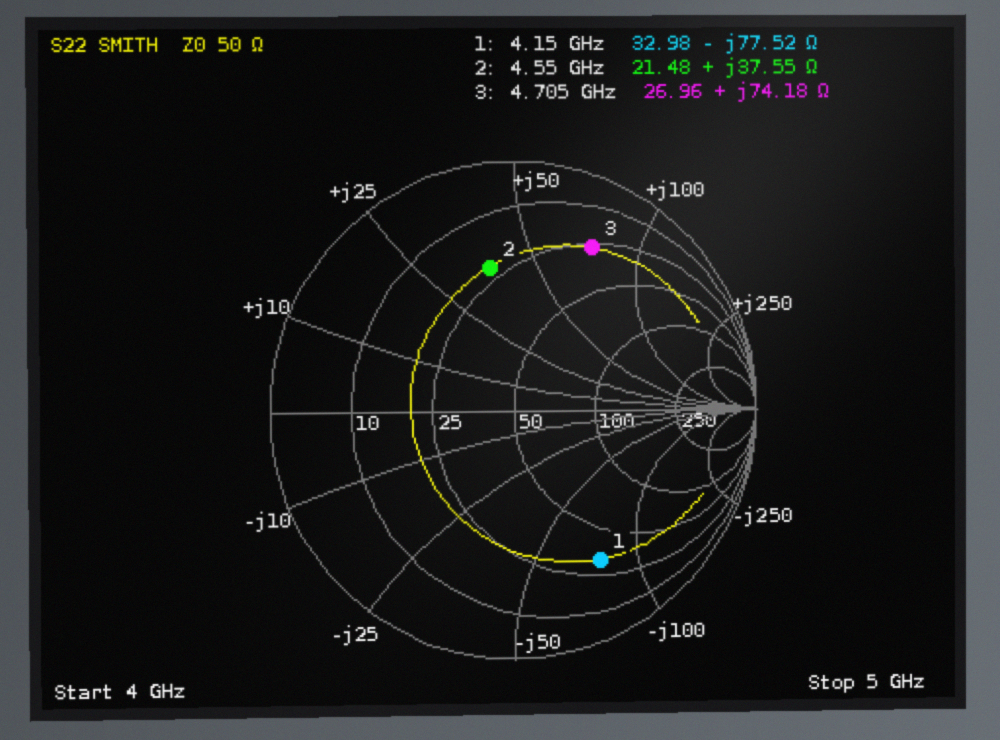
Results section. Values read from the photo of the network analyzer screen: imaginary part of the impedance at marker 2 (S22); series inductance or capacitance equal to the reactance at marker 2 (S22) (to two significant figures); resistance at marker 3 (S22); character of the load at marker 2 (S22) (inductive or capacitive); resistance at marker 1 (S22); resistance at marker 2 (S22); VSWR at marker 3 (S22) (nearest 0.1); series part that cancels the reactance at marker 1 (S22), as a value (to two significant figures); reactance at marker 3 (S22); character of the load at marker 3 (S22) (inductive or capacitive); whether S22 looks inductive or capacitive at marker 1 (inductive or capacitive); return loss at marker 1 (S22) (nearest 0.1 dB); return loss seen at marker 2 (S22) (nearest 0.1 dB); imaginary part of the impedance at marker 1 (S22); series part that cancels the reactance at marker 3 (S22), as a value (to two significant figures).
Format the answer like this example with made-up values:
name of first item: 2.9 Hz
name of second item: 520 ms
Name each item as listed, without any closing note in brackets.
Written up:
imaginary part of the impedance at marker 2: +37.55 Ω
series inductance or capacitance equal to the reactance at marker 2 (S22): 1.3 nH
resistance at marker 3: 26.96 Ω
character of the load at marker 2 (S22): inductive
resistance at marker 1: 32.98 Ω
resistance at marker 2: 21.48 Ω
VSWR at marker 3 (S22): 6.3
series part that cancels the reactance at marker 1 (S22), as a value: 3.0 nH
reactance at marker 3: +74.18 Ω
character of the load at marker 3 (S22): inductive
whether S22 looks inductive or capacitive at marker 1: capacitive
return loss at marker 1 (S22): 3.1 dB
return loss seen at marker 2 (S22): 4.7 dB
imaginary part of the impedance at marker 1: -77.52 Ω
series part that cancels the reactance at marker 3 (S22), as a value: 460 fF
